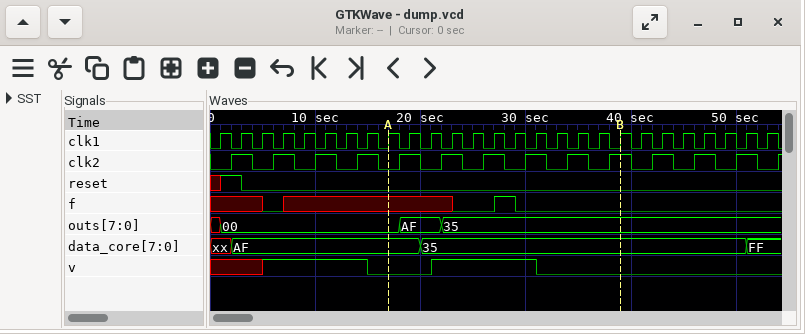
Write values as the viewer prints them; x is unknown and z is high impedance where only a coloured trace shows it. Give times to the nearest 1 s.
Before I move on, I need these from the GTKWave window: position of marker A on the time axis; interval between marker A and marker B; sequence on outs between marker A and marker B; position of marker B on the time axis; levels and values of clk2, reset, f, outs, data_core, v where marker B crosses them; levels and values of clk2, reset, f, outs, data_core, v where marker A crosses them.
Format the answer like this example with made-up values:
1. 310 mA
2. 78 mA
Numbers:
1. 17 s
2. 22 s
3. 00, AF, 35
4. 39 s
5. clk2=1, reset=0, f=0, outs=35, data_core=35, v=0
6. clk2=0, reset=0, f=x, outs=00, data_core=AF, v=0
